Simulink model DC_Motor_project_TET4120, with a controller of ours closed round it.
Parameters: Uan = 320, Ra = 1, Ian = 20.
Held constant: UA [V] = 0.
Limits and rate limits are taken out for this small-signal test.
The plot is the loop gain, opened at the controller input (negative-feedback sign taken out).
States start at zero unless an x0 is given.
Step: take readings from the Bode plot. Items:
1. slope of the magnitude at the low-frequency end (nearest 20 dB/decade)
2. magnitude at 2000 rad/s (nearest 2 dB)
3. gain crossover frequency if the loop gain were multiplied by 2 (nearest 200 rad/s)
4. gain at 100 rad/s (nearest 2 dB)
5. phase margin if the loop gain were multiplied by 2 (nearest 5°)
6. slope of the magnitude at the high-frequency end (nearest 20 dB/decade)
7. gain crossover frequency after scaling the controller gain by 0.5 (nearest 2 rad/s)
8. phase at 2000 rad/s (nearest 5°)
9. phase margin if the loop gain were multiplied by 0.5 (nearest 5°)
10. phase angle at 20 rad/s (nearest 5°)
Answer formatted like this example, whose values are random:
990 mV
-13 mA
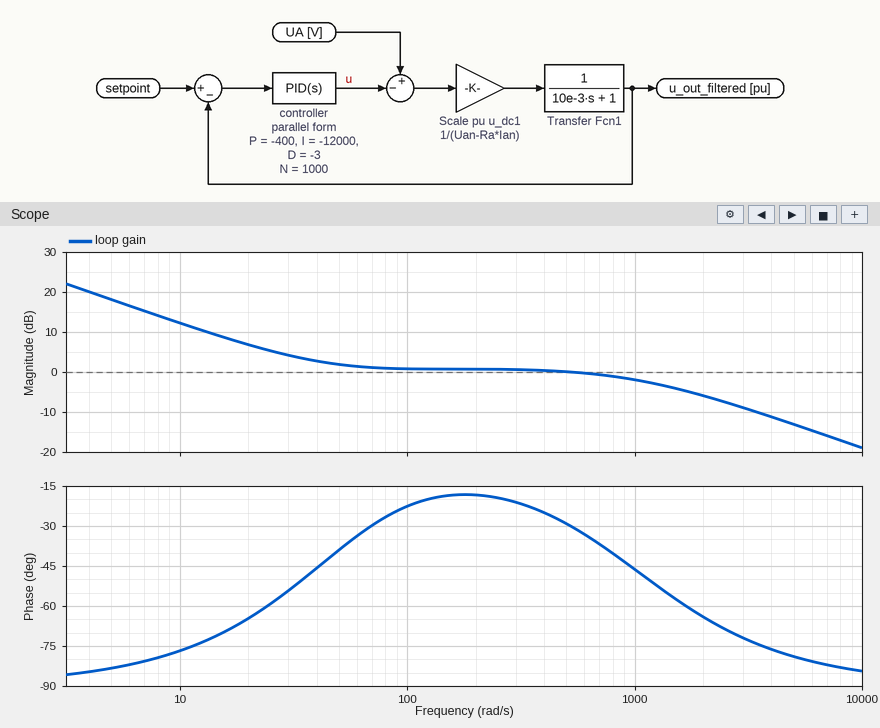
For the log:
-20 dB/decade
-6 dB
2000 rad/s
0 dB
115°
-20 dB/decade
22 rad/s
-65°
120°
-65°
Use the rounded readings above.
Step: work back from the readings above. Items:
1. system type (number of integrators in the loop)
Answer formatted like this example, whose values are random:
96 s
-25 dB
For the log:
1
